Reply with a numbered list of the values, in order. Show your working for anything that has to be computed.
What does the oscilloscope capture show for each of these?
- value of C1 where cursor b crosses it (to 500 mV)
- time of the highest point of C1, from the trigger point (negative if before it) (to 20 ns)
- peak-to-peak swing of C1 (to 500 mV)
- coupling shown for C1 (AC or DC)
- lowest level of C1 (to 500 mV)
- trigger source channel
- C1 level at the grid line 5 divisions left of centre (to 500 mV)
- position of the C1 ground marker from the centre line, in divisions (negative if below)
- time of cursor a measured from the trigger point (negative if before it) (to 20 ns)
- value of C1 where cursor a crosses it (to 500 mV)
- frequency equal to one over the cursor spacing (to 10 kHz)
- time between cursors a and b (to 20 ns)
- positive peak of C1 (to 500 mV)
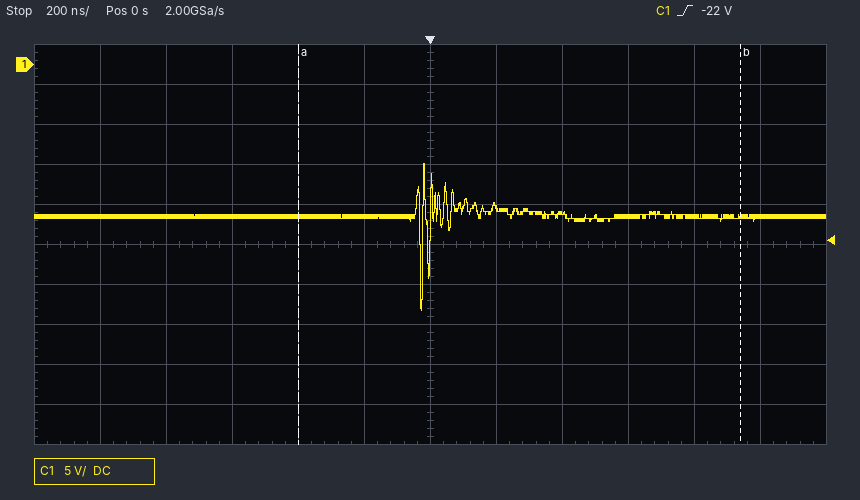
1. -19.0 V
2. -20 ns
3. -12.5 V − (-31.0 V) = 18.5 V
4. DC
5. -31.0 V
6. C1
7. -19.0 V
8. +4.5 div
9. -400 ns
10. -19.0 V
11. 1 / 1.34 µs ≈ 750 kHz
12. 1.34 µs
13. -12.5 V
